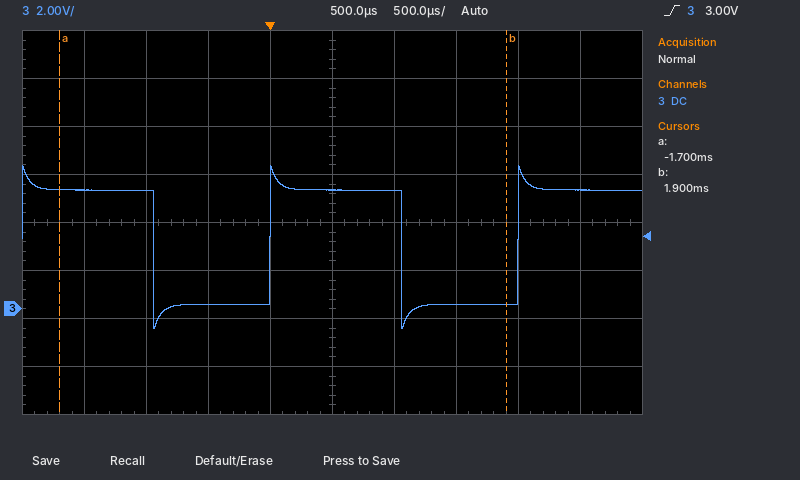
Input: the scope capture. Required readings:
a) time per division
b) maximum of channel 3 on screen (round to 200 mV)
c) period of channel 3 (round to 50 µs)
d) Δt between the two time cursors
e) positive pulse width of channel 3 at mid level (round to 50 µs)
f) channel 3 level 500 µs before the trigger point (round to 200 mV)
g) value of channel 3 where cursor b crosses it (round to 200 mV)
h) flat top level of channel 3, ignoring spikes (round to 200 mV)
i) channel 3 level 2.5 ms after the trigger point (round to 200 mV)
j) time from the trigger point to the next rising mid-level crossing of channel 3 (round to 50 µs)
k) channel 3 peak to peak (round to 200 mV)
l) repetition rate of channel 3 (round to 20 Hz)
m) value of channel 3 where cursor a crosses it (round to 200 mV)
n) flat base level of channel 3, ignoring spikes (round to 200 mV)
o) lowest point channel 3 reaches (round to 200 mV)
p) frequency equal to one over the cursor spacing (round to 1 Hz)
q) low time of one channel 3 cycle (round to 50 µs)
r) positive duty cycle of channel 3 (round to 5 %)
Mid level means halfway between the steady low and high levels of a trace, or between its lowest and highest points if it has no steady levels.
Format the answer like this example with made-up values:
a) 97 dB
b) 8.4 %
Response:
a) 500 µs
b) 6.0 V
c) 2.00 ms
d) 3.60 ms
e) 1.05 ms
f) 200 mV
g) 200 mV
h) 5.0 V
i) 5.0 V
j) 2.00 ms
k) 6.8 V
l) 500 Hz
m) 5.0 V
n) 200 mV
o) -800 mV
p) 278 Hz
q) 950 µs
r) 55 %
